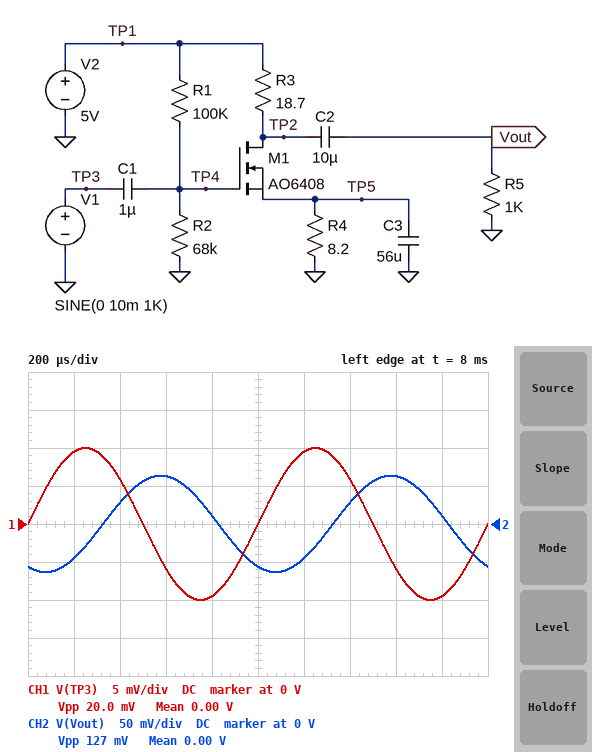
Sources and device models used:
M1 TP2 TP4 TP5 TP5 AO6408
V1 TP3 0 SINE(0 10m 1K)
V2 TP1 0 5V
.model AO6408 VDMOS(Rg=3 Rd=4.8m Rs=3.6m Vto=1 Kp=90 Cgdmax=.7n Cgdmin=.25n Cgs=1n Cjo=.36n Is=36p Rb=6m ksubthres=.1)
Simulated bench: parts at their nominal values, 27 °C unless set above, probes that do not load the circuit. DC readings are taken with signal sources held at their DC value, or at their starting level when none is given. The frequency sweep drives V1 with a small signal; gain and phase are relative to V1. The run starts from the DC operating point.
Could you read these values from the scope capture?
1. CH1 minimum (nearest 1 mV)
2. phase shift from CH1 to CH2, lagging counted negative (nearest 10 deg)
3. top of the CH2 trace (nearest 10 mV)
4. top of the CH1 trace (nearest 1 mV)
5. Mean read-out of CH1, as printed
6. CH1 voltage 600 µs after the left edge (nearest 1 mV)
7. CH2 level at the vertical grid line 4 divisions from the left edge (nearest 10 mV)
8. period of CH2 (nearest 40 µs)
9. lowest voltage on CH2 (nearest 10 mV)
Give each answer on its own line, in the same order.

-10 mV
-120 deg
60 mV
10 mV
0.00 V
-6 mV
10 mV
1.00 ms
-60 mV
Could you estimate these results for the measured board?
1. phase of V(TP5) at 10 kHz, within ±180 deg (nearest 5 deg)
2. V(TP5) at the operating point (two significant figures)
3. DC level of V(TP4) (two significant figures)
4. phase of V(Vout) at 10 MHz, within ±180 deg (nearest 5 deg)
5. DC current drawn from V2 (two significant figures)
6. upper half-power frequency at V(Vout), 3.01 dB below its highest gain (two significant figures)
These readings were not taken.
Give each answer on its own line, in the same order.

-60 deg
1.1 V
2.0 V
100 deg
130 mA
2.6 MHz
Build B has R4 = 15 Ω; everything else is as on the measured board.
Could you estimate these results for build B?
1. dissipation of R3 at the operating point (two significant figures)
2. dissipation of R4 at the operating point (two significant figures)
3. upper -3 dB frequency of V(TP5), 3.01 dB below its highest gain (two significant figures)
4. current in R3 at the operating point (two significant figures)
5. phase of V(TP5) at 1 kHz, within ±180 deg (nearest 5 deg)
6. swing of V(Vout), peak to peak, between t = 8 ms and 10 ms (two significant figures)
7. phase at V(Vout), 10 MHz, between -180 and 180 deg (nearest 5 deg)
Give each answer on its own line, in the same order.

99 mW
80 mW
3.6 kHz
73 mA
-15 deg
120 mV
110 deg
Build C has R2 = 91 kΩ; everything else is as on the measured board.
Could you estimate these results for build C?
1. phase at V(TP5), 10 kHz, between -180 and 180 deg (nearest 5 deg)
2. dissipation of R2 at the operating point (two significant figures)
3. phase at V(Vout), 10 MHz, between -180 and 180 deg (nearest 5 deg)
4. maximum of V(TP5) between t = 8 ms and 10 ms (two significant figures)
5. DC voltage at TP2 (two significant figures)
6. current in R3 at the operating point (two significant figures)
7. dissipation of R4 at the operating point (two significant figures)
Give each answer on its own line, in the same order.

-55 deg
62 µW
95 deg
1.4 V
1.8 V
170 mA
240 mW
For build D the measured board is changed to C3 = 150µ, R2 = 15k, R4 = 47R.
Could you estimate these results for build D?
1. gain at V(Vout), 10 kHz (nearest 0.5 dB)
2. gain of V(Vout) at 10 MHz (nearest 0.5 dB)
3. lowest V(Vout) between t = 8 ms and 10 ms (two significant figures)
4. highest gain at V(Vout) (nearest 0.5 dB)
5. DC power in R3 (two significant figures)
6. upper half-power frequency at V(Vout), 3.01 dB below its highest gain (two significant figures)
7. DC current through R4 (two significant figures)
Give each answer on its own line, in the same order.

-19.0 dB
-10.5 dB
-1.2 mV
-7.0 dB
1.8 µW
84 MHz
310 µA
